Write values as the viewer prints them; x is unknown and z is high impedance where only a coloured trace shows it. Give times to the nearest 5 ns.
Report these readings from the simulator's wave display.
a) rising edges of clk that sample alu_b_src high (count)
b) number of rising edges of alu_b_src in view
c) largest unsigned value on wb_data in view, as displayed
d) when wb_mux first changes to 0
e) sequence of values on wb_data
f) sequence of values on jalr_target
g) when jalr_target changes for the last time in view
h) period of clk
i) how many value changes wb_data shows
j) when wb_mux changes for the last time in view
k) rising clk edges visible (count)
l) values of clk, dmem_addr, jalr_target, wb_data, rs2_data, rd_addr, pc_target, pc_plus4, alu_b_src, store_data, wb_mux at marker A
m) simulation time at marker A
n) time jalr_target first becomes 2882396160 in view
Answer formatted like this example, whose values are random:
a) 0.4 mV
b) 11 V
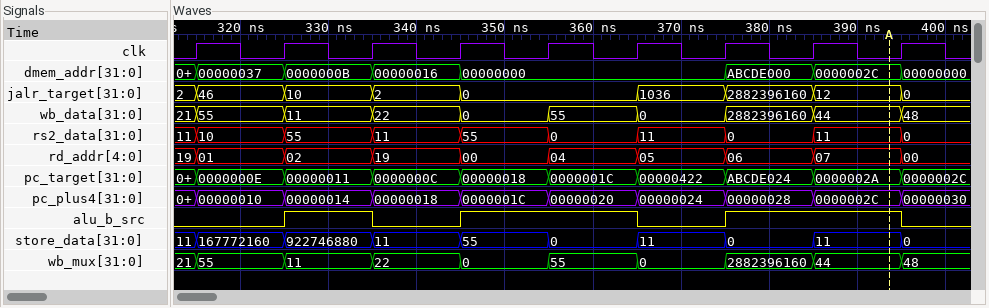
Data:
a) 5
b) 3
c) 2882396160
d) 345 ns
e) 21, 55, 11, 22, 0, 55, 0, 2882396160, 44, 48
f) 2, 46, 10, 2, 0, 1036, 2882396160, 12, 0
g) 395 ns
h) 10 ns
i) 9
j) 395 ns
k) 9
l) clk=0, dmem_addr=0000002C, jalr_target=12, wb_data=44, rs2_data=11, rd_addr=07, pc_target=0000002A, pc_plus4=0000002C, alu_b_src=1, store_data=11, wb_mux=44
m) 395 ns
n) 375 ns
